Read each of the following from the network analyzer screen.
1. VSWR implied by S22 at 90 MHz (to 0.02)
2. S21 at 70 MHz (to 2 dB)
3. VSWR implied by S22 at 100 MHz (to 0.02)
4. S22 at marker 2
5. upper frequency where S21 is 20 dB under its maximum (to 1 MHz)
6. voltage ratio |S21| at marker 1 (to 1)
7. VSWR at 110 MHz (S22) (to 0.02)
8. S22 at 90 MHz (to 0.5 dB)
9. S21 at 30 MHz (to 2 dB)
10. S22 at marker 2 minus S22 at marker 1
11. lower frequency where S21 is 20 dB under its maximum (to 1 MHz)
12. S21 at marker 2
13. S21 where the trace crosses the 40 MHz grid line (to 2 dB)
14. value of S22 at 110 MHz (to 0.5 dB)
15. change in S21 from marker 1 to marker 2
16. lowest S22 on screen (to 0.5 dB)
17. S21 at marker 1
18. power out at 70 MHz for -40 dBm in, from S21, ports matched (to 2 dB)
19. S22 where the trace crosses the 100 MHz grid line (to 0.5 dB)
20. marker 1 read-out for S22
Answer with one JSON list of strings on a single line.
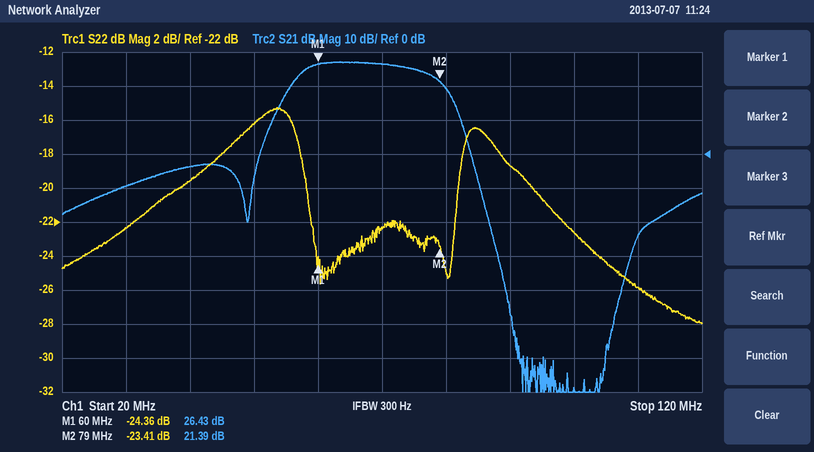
["1.26", "26 dB", "1.16", "-23.41 dB", "83 MHz", "21", "1.10", "-18.5 dB", "-10 dB", "0.95 dB", "52 MHz", "21.39 dB", "-4 dB", "-26.0 dB", "-5.04 dB", "-28.0 dB", "26.43 dB", "-14 dBm", "-22.5 dB", "-24.36 dB"]
